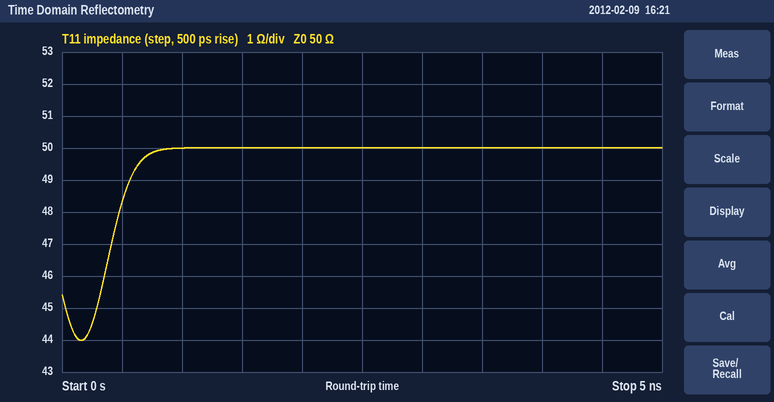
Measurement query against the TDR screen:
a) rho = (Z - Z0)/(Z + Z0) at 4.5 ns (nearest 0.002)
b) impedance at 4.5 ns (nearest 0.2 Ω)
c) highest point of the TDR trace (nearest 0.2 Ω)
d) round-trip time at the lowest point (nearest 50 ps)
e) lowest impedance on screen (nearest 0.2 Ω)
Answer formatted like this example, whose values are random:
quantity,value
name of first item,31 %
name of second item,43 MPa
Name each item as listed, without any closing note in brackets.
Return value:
quantity,value
rho = (Z - Z0)/(Z + Z0) at 4.5 ns,0.000
impedance at 4.5 ns,50.0 Ω
highest point of the TDR trace,50.0 Ω
round-trip time at the lowest point,150 ps
lowest impedance on screen,44.0 Ω
